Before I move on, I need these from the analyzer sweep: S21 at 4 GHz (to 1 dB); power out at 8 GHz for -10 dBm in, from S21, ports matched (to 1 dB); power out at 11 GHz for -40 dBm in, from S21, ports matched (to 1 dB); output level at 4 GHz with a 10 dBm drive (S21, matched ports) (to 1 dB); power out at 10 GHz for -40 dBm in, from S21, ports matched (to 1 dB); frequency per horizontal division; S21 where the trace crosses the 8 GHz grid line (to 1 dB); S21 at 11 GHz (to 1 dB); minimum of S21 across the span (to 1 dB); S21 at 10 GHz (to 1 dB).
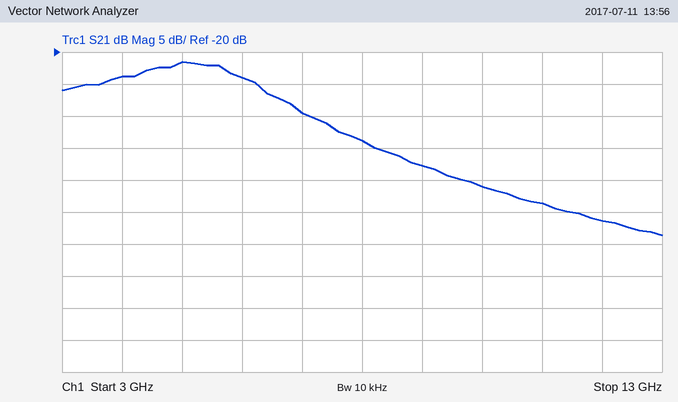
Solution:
-24 dB
-44 dBm
-84 dBm
-14 dBm
-81 dBm
1 GHz
-34 dB
-44 dB
-49 dB
-41 dB
